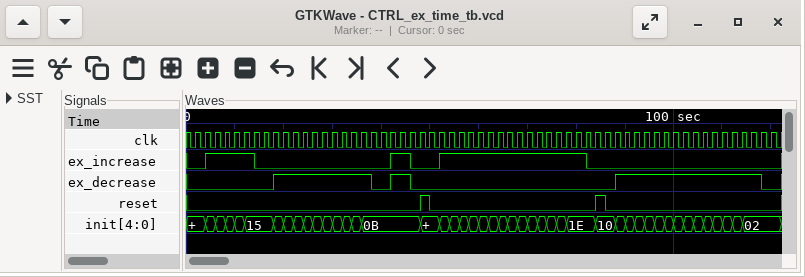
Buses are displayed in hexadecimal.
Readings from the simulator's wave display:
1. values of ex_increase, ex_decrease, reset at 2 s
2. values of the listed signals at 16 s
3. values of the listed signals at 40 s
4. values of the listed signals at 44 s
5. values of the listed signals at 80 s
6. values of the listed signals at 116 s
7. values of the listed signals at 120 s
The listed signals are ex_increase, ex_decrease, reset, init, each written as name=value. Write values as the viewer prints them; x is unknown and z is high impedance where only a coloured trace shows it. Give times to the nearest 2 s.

ex_increase=0, ex_decrease=0, reset=0
ex_increase=0, ex_decrease=0, reset=0, init=15
ex_increase=0, ex_decrease=0, reset=0, init=0B
ex_increase=1, ex_decrease=1, reset=0, init=0B
ex_increase=1, ex_decrease=0, reset=0, init=1E
ex_increase=0, ex_decrease=1, reset=0, init=02
ex_increase=0, ex_decrease=0, reset=0, init=02
